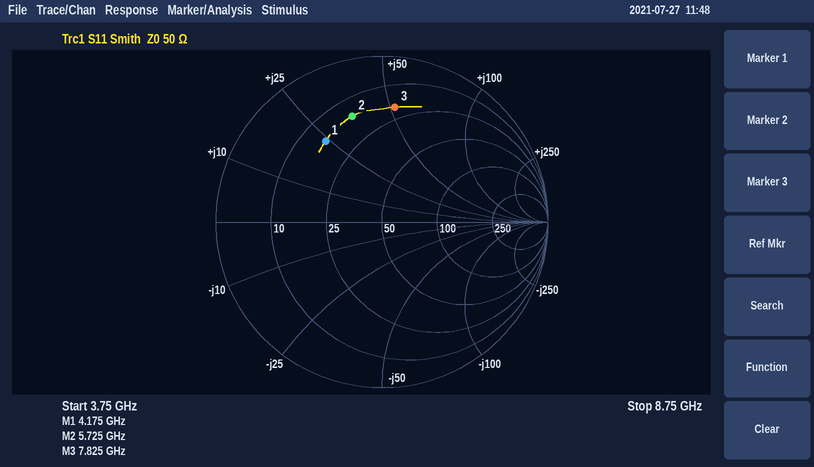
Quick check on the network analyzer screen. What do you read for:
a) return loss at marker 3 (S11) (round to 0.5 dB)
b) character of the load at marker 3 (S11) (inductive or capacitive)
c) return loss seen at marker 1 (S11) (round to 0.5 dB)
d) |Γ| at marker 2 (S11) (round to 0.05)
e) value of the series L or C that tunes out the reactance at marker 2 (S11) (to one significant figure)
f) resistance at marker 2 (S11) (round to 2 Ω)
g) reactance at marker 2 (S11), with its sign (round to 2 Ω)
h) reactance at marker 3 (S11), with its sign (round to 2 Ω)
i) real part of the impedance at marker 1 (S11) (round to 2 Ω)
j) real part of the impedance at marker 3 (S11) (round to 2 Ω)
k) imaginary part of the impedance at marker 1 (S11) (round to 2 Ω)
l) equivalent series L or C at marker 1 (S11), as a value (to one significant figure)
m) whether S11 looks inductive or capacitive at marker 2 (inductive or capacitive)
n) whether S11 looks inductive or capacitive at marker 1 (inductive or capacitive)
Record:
3.0 dB
inductive
4.5 dB
0.65
800 fF
16 Ω
+36 Ω
+52 Ω
16 Ω
20 Ω
+24 Ω
900 pH
inductive
inductive
